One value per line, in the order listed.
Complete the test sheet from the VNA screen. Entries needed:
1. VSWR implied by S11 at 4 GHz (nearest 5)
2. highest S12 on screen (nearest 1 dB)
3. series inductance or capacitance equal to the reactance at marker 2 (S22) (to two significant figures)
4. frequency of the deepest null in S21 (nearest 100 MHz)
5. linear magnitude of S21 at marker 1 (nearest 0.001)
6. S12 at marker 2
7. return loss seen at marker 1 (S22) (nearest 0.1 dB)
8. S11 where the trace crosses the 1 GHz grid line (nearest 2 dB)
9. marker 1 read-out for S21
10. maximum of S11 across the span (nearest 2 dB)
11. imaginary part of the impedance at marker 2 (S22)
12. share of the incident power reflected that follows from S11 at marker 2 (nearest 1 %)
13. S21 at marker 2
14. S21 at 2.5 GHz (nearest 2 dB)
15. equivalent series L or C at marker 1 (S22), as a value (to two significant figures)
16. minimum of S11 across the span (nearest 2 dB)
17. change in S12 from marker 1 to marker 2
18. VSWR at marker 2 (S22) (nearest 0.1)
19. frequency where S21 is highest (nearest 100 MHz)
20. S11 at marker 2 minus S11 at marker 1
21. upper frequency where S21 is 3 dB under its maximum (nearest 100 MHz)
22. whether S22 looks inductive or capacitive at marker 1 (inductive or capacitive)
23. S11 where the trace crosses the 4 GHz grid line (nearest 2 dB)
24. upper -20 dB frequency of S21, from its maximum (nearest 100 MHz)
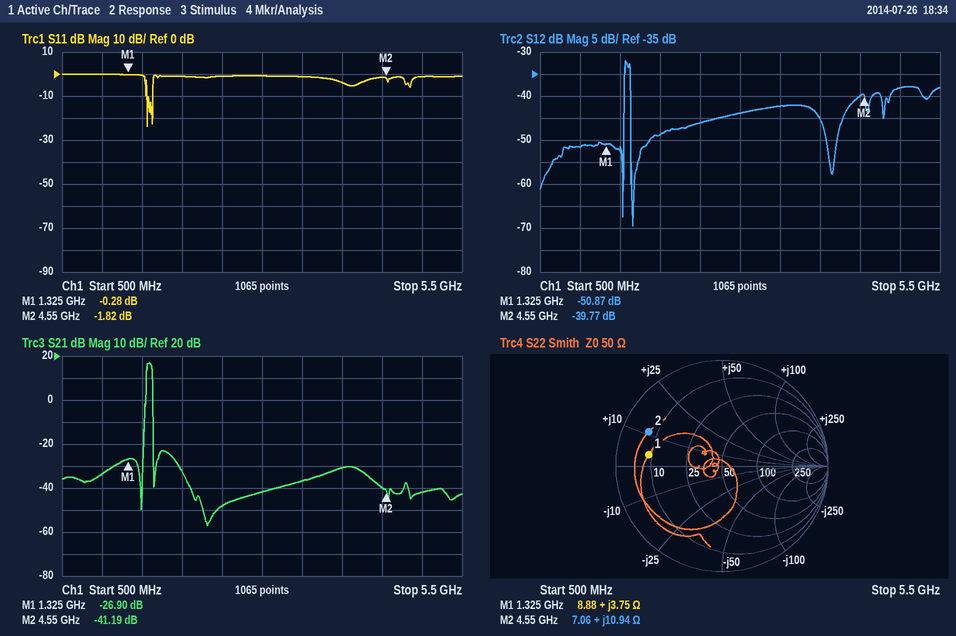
5
-32 dB
380 pH
2.3 GHz
0.045
-39.77 dB
3.1 dB
0 dB
-26.90 dB
0 dB
+10.94 Ω
66 %
-41.19 dB
-48 dB
450 pH
-24 dB
11.10 dB
7.4
1.6 GHz
-1.54 dB
1.6 GHz
inductive
-4 dB
1.6 GHz
